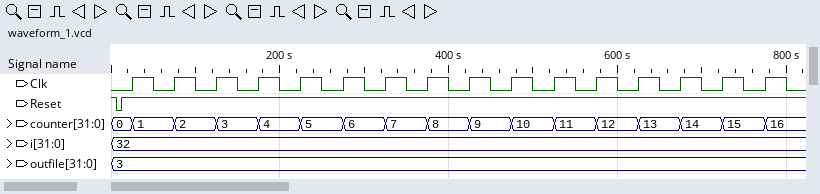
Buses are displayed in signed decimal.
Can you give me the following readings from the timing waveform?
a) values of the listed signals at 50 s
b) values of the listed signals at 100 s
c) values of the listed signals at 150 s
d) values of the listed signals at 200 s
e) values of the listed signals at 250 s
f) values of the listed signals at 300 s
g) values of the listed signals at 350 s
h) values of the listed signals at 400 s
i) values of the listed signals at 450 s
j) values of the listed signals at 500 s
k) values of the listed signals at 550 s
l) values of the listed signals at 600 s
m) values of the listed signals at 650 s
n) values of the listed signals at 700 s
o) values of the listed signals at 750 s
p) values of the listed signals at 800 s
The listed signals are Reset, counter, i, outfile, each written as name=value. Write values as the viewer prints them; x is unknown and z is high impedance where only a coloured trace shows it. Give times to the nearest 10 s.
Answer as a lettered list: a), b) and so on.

a) Reset=1, counter=1, i=32, outfile=3
b) Reset=1, counter=2, i=32, outfile=3
c) Reset=1, counter=3, i=32, outfile=3
d) Reset=1, counter=4, i=32, outfile=3
e) Reset=1, counter=5, i=32, outfile=3
f) Reset=1, counter=6, i=32, outfile=3
g) Reset=1, counter=7, i=32, outfile=3
h) Reset=1, counter=8, i=32, outfile=3
i) Reset=1, counter=9, i=32, outfile=3
j) Reset=1, counter=10, i=32, outfile=3
k) Reset=1, counter=11, i=32, outfile=3
l) Reset=1, counter=12, i=32, outfile=3
m) Reset=1, counter=13, i=32, outfile=3
n) Reset=1, counter=14, i=32, outfile=3
o) Reset=1, counter=15, i=32, outfile=3
p) Reset=1, counter=16, i=32, outfile=3
